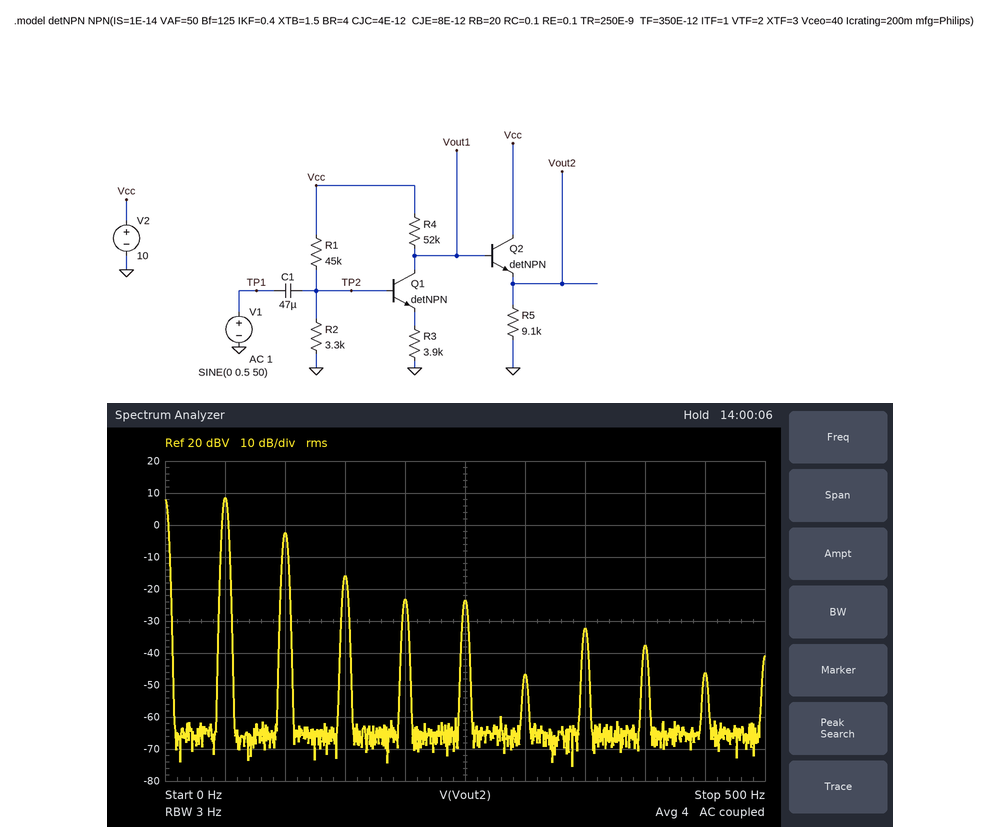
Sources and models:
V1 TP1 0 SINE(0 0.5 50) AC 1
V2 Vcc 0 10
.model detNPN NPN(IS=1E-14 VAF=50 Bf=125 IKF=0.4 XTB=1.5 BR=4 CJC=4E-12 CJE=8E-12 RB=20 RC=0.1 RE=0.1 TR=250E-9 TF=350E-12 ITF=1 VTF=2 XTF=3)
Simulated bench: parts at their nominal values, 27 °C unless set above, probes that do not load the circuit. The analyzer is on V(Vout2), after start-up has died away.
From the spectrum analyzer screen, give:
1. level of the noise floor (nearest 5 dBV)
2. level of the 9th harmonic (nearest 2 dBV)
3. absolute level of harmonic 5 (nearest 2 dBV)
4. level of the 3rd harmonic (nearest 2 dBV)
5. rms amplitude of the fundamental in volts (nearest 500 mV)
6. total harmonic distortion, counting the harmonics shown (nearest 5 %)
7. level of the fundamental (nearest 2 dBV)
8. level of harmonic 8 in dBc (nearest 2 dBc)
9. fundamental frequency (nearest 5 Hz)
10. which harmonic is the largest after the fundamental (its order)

-65 dBV
-46 dBV
-24 dBV
-16 dBV
2.5 V
30 %
8 dBV
-46 dBc
50 Hz
2
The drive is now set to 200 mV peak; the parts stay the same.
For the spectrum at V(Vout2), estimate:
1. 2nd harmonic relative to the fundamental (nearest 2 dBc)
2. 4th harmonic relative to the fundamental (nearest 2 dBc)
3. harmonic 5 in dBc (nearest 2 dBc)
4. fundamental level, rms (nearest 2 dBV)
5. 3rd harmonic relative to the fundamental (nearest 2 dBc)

-20 dBc
-42 dBc
-58 dBc
2 dBV
-30 dBc
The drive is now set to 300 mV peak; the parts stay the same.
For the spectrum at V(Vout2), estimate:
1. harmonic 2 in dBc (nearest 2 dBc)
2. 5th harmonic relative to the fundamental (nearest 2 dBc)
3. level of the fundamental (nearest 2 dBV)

-14 dBc
-42 dBc
6 dBV
